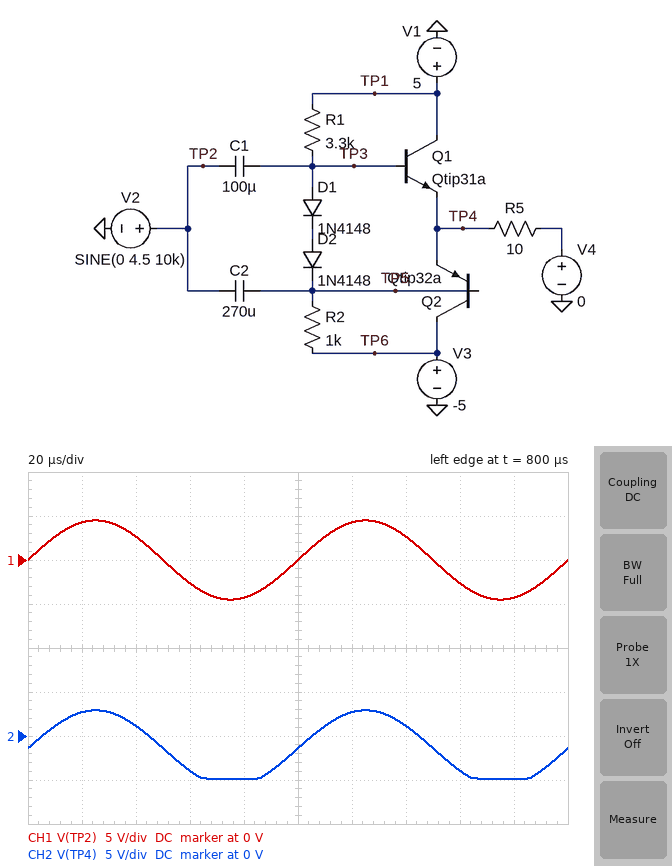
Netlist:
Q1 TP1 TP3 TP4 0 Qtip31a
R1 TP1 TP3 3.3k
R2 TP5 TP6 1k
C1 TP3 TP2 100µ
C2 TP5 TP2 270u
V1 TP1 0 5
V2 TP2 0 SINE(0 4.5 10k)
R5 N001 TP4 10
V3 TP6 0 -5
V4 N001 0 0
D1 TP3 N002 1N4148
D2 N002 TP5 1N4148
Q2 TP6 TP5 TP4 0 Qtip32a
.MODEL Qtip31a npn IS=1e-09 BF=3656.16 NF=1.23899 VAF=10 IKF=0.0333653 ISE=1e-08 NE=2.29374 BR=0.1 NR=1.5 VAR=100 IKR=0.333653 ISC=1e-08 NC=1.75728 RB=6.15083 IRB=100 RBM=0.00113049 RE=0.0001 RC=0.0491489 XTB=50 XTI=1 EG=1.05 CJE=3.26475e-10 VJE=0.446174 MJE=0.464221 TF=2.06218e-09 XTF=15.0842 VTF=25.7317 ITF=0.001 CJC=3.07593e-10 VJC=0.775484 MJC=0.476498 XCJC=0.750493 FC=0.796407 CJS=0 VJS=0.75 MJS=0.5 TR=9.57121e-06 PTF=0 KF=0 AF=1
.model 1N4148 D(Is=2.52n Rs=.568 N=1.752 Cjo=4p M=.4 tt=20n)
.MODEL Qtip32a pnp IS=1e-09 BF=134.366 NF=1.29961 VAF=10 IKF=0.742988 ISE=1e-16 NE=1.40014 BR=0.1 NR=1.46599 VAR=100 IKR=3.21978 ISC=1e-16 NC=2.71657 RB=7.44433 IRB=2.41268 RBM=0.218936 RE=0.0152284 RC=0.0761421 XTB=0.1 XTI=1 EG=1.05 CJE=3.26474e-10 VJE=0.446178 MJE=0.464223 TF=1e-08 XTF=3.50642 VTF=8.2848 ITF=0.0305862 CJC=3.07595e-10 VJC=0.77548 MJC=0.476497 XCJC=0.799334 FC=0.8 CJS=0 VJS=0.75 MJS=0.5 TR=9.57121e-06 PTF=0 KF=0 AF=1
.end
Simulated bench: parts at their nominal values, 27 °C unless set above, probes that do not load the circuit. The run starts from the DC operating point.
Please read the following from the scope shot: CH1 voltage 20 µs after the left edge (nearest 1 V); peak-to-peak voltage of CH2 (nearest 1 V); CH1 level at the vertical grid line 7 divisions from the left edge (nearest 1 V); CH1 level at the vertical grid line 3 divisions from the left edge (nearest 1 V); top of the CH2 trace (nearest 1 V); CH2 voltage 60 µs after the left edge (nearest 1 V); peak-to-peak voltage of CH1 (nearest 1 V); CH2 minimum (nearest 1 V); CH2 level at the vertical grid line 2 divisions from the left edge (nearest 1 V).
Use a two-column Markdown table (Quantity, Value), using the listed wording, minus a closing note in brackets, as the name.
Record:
| Quantity | Value |
|---|---|
| CH1 voltage 20 µs after the left edge | 4 V |
| peak-to-peak voltage of CH2 | 8 V |
| CH1 level at the vertical grid line 7 divisions from the left edge | 3 V |
| CH1 level at the vertical grid line 3 divisions from the left edge | -3 V |
| top of the CH2 trace | 3 V |
| CH2 voltage 60 µs after the left edge | -4 V |
| peak-to-peak voltage of CH1 | 9 V |
| CH2 minimum | -5 V |
| CH2 level at the vertical grid line 2 divisions from the left edge | 1 V |
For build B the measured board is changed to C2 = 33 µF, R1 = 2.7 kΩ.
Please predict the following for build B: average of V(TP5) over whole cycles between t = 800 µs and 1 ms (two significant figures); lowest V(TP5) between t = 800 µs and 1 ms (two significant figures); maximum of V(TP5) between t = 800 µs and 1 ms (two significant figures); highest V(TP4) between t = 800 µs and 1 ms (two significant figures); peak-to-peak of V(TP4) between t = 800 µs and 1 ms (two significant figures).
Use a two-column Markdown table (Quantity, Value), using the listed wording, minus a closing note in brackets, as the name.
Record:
| Quantity | Value |
|---|---|
| average of V(TP5) over whole cycles between t = 800 µs and 1 ms | -1.6 V |
| lowest V(TP5) between t = 800 µs and 1 ms | -6.1 V |
| maximum of V(TP5) between t = 800 µs and 1 ms | 2.9 V |
| highest V(TP4) between t = 800 µs and 1 ms | 3.1 V |
| peak-to-peak of V(TP4) between t = 800 µs and 1 ms | 8.0 V |
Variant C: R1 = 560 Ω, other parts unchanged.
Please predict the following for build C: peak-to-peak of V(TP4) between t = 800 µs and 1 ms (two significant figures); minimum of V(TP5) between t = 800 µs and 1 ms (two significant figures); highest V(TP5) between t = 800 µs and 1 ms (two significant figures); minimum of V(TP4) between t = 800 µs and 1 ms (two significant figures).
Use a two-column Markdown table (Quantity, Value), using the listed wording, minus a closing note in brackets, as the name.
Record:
| Quantity | Value |
|---|---|
| peak-to-peak of V(TP4) between t = 800 µs and 1 ms | 8.2 V |
| minimum of V(TP5) between t = 800 µs and 1 ms | -4.1 V |
| highest V(TP5) between t = 800 µs and 1 ms | 4.9 V |
| minimum of V(TP4) between t = 800 µs and 1 ms | -3.4 V |
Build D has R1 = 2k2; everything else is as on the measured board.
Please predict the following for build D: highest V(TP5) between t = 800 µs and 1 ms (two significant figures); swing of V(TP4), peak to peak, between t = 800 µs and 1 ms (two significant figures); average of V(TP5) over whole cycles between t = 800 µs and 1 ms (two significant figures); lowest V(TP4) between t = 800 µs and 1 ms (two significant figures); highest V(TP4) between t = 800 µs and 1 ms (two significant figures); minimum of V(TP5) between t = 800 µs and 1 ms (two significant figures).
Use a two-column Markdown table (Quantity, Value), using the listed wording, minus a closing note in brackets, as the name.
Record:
| Quantity | Value |
|---|---|
| highest V(TP5) between t = 800 µs and 1 ms | 2.9 V |
| swing of V(TP4), peak to peak, between t = 800 µs and 1 ms | 8.2 V |
| average of V(TP5) over whole cycles between t = 800 µs and 1 ms | -1.6 V |
| lowest V(TP4) between t = 800 µs and 1 ms | -4.9 V |
| highest V(TP4) between t = 800 µs and 1 ms | 3.4 V |
| minimum of V(TP5) between t = 800 µs and 1 ms | -6.1 V |
